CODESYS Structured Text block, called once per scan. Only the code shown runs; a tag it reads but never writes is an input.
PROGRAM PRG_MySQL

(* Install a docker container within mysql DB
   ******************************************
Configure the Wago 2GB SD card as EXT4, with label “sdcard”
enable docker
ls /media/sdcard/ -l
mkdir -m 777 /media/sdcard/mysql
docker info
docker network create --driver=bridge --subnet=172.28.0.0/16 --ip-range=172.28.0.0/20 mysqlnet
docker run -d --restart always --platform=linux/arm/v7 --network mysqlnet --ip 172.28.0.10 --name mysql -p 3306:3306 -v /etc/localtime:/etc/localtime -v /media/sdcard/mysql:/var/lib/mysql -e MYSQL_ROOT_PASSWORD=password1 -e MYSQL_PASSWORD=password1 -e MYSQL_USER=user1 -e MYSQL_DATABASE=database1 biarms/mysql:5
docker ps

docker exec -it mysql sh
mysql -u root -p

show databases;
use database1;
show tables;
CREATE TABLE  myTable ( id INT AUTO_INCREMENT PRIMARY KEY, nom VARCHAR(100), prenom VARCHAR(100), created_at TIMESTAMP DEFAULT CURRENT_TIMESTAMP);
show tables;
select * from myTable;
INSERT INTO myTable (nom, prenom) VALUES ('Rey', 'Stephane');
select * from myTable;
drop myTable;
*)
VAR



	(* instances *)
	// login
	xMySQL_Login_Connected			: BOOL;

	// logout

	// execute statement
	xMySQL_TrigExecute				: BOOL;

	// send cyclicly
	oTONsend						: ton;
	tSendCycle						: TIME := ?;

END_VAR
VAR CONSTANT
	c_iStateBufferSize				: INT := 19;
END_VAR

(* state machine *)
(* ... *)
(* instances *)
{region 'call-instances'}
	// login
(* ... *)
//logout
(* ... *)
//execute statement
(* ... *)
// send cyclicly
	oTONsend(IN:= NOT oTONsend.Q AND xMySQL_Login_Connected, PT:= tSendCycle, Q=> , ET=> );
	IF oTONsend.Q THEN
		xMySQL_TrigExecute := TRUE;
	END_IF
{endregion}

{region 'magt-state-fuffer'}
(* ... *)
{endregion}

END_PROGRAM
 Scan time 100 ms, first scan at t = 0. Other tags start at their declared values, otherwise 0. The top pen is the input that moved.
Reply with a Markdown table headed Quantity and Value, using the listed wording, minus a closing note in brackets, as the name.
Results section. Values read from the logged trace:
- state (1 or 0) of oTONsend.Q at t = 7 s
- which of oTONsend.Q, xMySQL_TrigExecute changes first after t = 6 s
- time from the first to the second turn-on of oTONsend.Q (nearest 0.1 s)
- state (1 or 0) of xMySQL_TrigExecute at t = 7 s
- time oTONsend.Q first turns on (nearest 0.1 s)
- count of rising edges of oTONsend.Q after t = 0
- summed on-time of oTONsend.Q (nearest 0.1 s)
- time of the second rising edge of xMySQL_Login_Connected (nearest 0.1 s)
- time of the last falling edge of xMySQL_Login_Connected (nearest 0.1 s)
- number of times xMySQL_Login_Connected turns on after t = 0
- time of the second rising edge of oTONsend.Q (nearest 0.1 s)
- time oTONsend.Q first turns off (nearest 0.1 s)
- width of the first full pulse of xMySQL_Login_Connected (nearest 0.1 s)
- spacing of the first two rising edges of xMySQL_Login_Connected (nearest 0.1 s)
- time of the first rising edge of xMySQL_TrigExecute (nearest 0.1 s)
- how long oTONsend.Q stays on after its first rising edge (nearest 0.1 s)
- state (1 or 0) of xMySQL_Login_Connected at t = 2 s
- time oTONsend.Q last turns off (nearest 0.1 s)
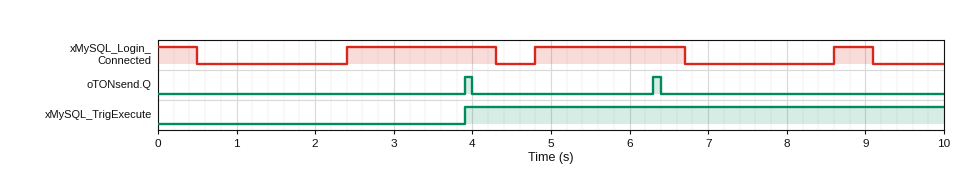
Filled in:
| Quantity | Value |
|---|---|
| state (1 or 0) of oTONsend.Q at t = 7 s | 0 |
| which of oTONsend.Q, xMySQL_TrigExecute changes first after t = 6 s | oTONsend.Q |
| time from the first to the second turn-on of oTONsend.Q | 2.4 s |
| state (1 or 0) of xMySQL_TrigExecute at t = 7 s | 1 |
| time oTONsend.Q first turns on | 3.9 s |
| count of rising edges of oTONsend.Q after t = 0 | 2 |
| summed on-time of oTONsend.Q | 0.2 s |
| time of the second rising edge of xMySQL_Login_Connected | 4.8 s |
| time of the last falling edge of xMySQL_Login_Connected | 9.1 s |
| number of times xMySQL_Login_Connected turns on after t = 0 | 3 |
| time of the second rising edge of oTONsend.Q | 6.3 s |
| time oTONsend.Q first turns off | 4.0 s |
| width of the first full pulse of xMySQL_Login_Connected | 1.9 s |
| spacing of the first two rising edges of xMySQL_Login_Connected | 2.4 s |
| time of the first rising edge of xMySQL_TrigExecute | 3.9 s |
| how long oTONsend.Q stays on after its first rising edge | 0.1 s |
| state (1 or 0) of xMySQL_Login_Connected at t = 2 s | 0 |
| time oTONsend.Q last turns off | 6.4 s |
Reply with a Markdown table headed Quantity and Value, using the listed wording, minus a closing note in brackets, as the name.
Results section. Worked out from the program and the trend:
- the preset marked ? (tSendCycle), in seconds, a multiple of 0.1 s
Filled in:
| Quantity | Value |
|---|---|
| the preset marked ? (tSendCycle), in seconds, a multiple of 0.1 s | 1.5 s |
